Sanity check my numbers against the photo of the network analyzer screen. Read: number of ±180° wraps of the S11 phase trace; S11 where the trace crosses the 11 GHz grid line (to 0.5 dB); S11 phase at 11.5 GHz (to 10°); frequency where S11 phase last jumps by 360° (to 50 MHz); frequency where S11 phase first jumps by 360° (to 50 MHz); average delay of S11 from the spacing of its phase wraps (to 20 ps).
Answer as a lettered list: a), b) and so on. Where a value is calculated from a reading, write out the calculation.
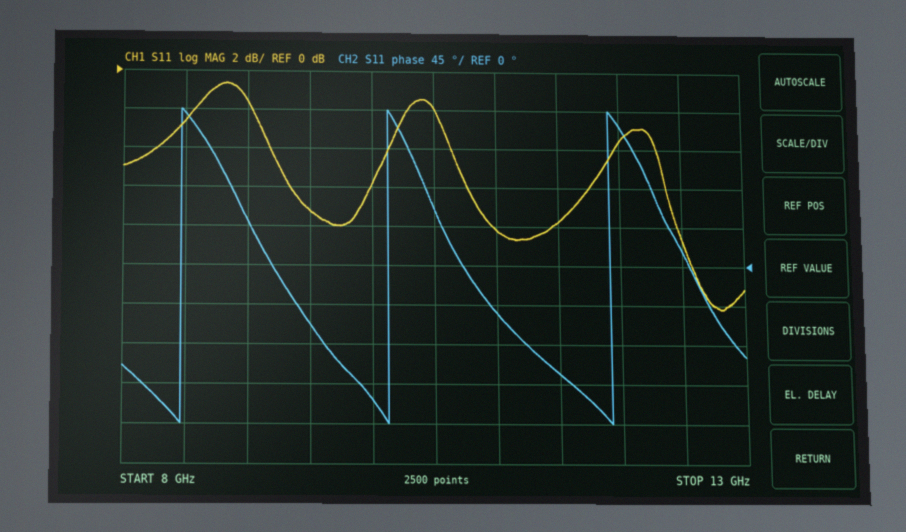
a) 3
b) -8.0 dB
c) -120°
d) 11.90 GHz
e) 8.45 GHz
f) 2 cycles / (11.90 GHz − 8.45 GHz) ≈ 580 ps
